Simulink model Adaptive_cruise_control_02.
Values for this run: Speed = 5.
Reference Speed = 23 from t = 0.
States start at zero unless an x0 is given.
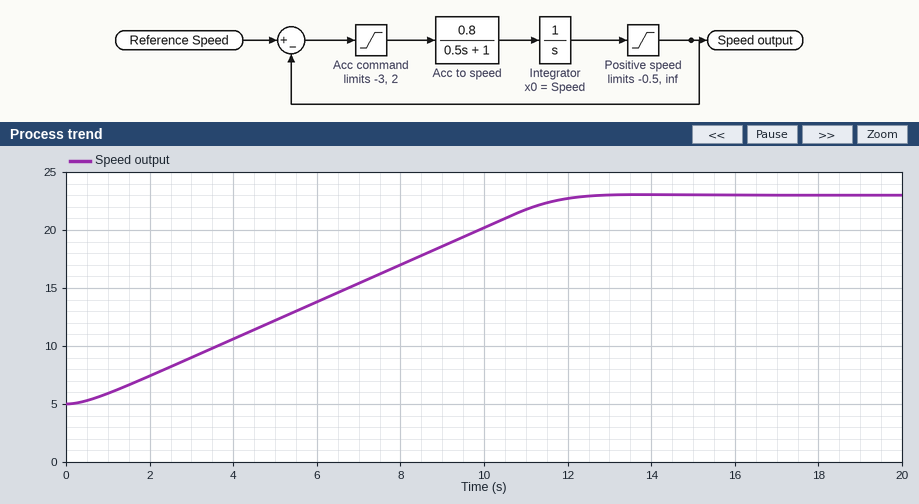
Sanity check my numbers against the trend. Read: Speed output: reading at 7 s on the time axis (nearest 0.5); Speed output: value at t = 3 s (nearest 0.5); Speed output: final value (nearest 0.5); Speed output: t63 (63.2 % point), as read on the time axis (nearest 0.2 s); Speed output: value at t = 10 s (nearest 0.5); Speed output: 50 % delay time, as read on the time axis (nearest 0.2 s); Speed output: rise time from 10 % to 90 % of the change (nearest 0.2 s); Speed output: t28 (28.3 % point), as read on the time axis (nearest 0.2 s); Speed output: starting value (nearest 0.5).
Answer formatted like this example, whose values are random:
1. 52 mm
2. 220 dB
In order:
1. 15.5
2. 9.0
3. 23.0
4. 7.6 s
5. 20.0
6. 6.2 s
7. 9.0 s
8. 3.6 s
9. 5.0
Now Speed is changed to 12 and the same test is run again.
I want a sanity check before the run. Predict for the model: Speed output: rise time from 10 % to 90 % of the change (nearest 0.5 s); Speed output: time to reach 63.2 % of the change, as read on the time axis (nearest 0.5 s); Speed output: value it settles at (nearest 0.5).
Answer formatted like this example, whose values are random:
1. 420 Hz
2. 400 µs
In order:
1. 5.5 s
2. 5.0 s
3. 23.0
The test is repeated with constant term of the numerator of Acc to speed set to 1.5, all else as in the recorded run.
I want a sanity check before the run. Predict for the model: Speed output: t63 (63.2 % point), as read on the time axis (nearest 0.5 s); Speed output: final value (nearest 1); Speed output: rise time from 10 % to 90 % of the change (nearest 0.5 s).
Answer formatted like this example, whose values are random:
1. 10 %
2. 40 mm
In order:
1. 4.5 s
2. 23
3. 5.0 s
